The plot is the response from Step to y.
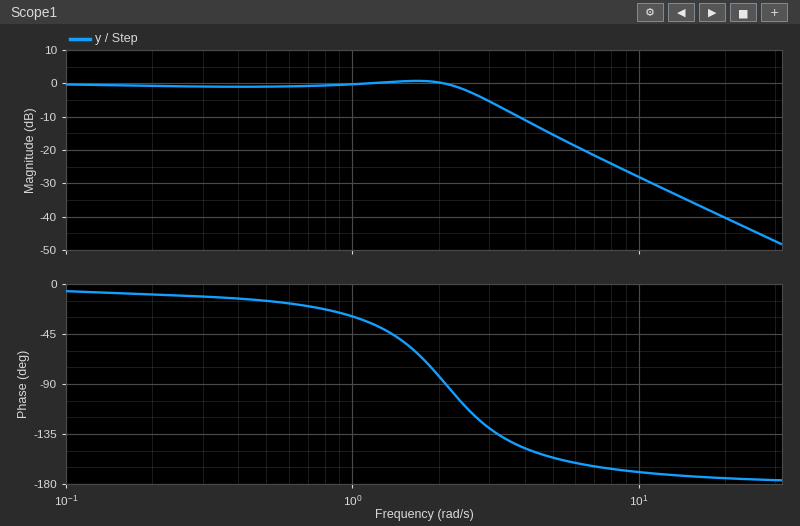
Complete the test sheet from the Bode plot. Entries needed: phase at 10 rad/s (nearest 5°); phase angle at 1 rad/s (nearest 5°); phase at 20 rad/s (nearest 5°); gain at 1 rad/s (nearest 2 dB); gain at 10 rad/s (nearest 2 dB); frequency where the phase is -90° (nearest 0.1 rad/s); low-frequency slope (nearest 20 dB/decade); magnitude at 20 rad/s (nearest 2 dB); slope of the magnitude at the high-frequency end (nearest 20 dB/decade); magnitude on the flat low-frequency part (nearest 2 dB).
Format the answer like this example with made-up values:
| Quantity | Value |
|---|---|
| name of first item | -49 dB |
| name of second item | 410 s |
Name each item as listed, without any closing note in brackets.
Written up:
| Quantity | Value |
|---|---|
| phase at 10 rad/s | -170° |
| phase angle at 1 rad/s | -30° |
| phase at 20 rad/s | -175° |
| gain at 1 rad/s | 0 dB |
| gain at 10 rad/s | -28 dB |
| frequency where the phase is -90° | 2.1 rad/s |
| low-frequency slope | 0 dB/decade |
| magnitude at 20 rad/s | -40 dB |
| slope of the magnitude at the high-frequency end | -40 dB/decade |
| magnitude on the flat low-frequency part | 0 dB |
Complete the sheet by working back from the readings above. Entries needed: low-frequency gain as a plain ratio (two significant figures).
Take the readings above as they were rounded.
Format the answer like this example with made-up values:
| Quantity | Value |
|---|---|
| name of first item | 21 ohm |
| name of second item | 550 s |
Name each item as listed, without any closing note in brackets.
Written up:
| Quantity | Value |
|---|---|
| low-frequency gain as a plain ratio | 1.0 |
